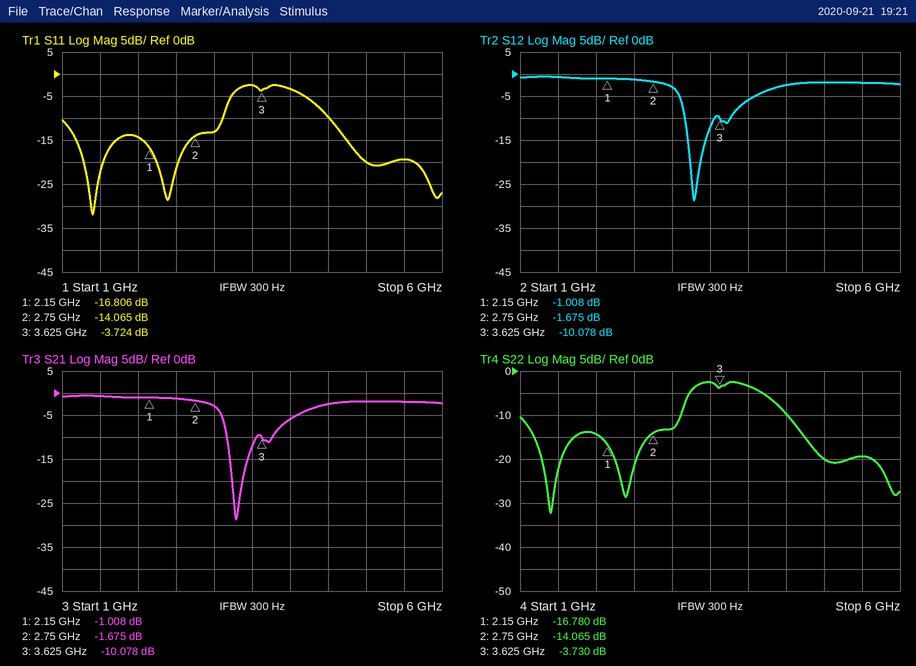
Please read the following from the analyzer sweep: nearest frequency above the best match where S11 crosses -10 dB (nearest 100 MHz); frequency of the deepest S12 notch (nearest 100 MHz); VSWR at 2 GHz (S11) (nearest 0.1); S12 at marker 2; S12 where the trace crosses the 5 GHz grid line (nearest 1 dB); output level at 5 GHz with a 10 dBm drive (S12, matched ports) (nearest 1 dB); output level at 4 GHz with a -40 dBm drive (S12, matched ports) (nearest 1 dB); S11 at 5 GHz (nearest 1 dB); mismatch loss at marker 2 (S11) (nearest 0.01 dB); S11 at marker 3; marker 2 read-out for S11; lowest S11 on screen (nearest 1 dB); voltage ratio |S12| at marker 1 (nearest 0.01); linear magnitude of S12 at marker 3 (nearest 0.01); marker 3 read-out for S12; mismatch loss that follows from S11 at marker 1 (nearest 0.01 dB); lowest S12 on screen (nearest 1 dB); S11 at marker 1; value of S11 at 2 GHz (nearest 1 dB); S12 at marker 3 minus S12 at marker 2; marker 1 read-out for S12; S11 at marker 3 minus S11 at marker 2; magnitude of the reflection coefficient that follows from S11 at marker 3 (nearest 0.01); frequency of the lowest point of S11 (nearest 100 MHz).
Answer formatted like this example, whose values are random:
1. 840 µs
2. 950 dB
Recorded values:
1. 3.1 GHz
2. 3.3 GHz
3. 1.5
4. -1.675 dB
5. -2 dB
6. 8 dBm
7. -46 dBm
8. -20 dB
9. 0.17 dB
10. -3.724 dB
11. -14.065 dB
12. -32 dB
13. 0.89
14. 0.31
15. -10.078 dB
16. 0.09 dB
17. -29 dB
18. -16.806 dB
19. -14 dB
20. -8.403 dB
21. -1.008 dB
22. 10.341 dB
23. 0.65
24. 1.4 GHz
